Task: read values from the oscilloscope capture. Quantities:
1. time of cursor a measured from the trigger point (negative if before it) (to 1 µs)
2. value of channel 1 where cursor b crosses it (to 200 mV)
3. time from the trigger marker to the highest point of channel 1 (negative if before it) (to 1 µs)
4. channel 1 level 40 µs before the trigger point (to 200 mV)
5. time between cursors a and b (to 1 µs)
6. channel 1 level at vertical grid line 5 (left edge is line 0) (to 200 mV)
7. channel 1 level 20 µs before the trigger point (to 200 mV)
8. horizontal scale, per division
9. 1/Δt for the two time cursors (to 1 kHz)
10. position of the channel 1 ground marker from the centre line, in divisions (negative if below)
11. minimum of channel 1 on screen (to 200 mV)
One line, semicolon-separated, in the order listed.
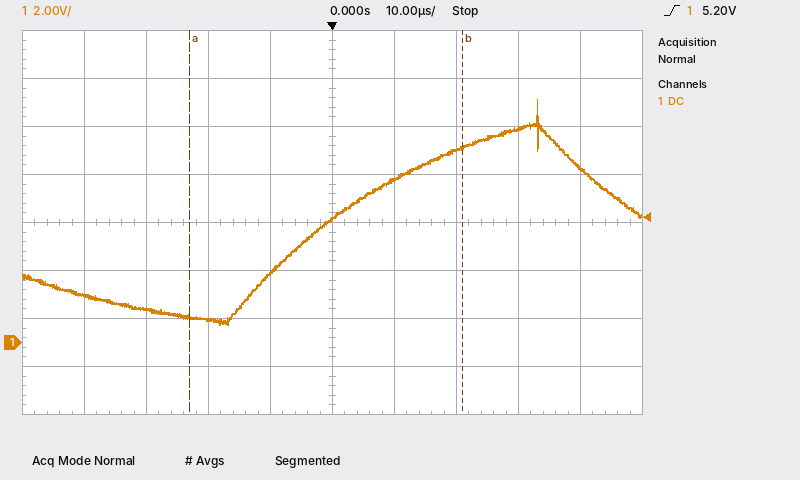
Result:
-23 µs; 8.2 V; +33 µs; 2.0 V; 44 µs; 5.2 V; 1.0 V; 10 µs; 23 kHz; -2.5 div; 800 mV
